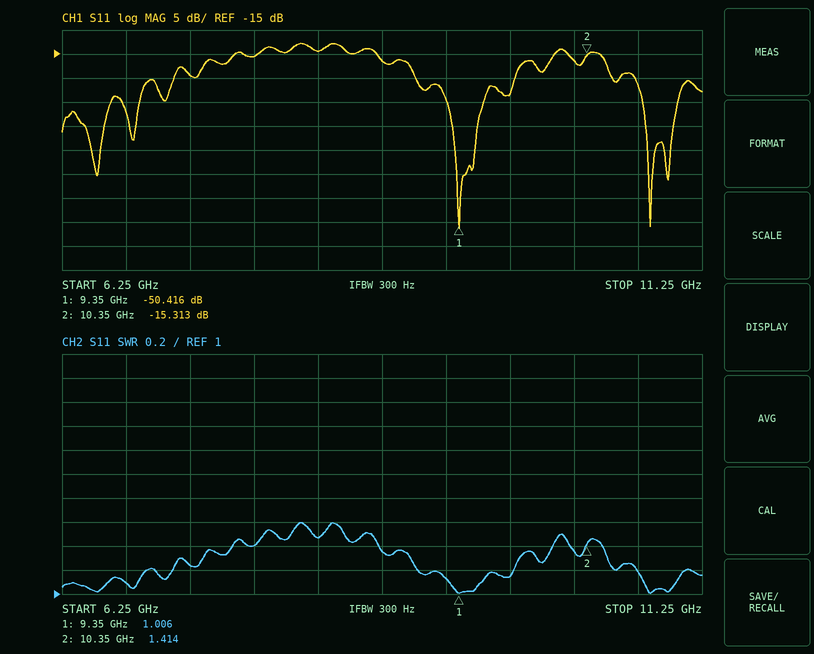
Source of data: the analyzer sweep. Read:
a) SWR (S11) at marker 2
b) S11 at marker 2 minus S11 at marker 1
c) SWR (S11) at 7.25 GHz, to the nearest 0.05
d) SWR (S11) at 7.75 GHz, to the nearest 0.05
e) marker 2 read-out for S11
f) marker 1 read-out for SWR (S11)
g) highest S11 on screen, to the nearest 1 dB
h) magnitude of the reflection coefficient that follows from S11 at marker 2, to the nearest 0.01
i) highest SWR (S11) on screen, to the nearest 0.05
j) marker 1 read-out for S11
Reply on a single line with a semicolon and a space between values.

1.414; 35.103 dB; 1.25; 1.40; -15.313 dB; 1.006; -13 dB; 0.17; 1.60; -50.416 dB
